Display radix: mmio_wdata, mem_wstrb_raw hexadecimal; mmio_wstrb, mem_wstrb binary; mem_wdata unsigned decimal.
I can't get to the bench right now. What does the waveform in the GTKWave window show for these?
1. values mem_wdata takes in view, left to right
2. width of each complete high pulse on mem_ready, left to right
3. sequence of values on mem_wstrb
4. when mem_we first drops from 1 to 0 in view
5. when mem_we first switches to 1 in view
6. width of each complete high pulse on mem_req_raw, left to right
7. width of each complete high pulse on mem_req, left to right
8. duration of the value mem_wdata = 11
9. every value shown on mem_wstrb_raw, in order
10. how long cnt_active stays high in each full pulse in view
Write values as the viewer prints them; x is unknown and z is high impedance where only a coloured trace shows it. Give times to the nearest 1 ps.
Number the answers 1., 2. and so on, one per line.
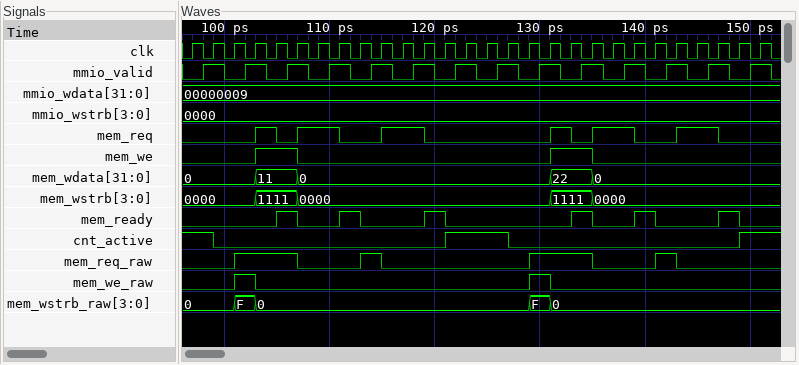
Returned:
1. 0, 11, 0, 22, 0
2. 2 ps, 2 ps, 2 ps, 2 ps, 2 ps, 2 ps
3. 0000, 1111, 0000, 1111, 0000
4. 107 ps
5. 103 ps
6. 6 ps, 2 ps, 6 ps, 2 ps
7. 2 ps, 4 ps, 4 ps, 2 ps, 4 ps, 4 ps
8. 4 ps
9. 0, F, 0, F, 0
10. 6 ps
